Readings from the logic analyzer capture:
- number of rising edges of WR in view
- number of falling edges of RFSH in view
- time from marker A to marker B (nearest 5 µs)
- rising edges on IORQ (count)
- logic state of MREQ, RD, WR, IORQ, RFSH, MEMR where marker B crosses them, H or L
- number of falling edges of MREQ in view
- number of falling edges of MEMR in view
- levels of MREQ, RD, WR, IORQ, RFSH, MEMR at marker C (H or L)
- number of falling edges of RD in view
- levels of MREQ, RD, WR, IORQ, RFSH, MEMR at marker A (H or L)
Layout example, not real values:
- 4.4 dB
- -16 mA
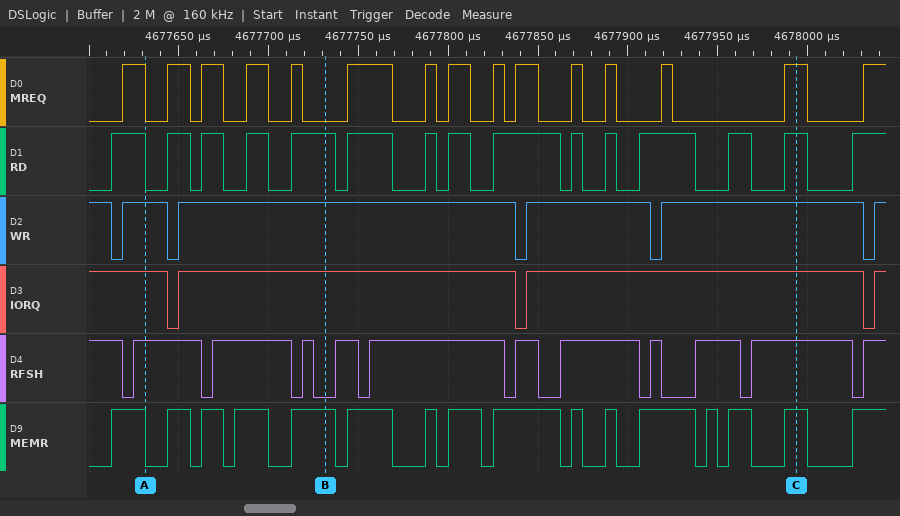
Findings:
- 5
- 11
- 100 µs
- 3
- MREQ=L, RD=H, WR=H, IORQ=H, RFSH=L, MEMR=H
- 14
- 15
- MREQ=H, RD=H, WR=H, IORQ=H, RFSH=H, MEMR=H
- 14
- MREQ=L, RD=L, WR=H, IORQ=H, RFSH=H, MEMR=L
